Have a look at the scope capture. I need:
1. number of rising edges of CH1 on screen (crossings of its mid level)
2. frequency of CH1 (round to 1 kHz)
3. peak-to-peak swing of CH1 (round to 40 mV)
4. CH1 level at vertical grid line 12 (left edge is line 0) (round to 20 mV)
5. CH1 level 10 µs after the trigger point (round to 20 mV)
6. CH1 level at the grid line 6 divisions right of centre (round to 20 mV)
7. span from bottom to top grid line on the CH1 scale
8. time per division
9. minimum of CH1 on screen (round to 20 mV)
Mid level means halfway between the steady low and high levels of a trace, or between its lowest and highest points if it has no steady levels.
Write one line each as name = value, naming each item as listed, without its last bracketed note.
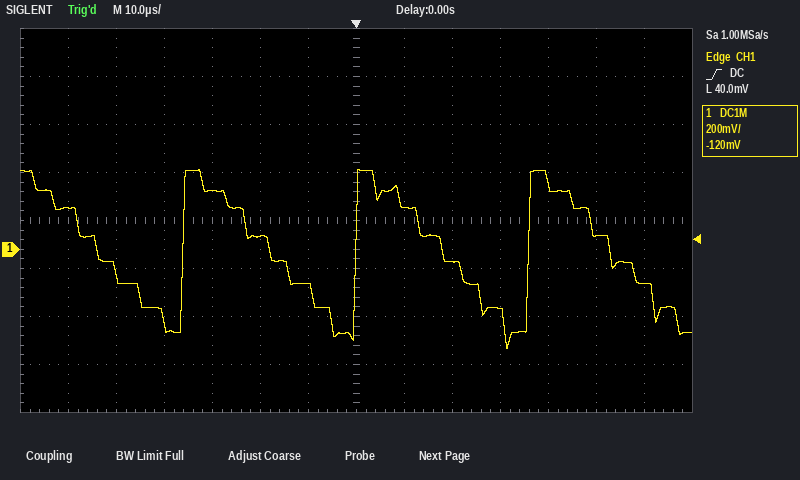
number of rising edges of CH1 on screen = 3
frequency of CH1 = 28 kHz
peak-to-peak swing of CH1 = 760 mV
CH1 level at vertical grid line 12 (left edge is line 0) = 60 mV
CH1 level 10 µs after the trigger point = 180 mV
CH1 level at the grid line 6 divisions right of centre = -140 mV
span from bottom to top grid line on the CH1 scale = 1.6 V
time per division = 10 µs
minimum of CH1 on screen = -420 mV
